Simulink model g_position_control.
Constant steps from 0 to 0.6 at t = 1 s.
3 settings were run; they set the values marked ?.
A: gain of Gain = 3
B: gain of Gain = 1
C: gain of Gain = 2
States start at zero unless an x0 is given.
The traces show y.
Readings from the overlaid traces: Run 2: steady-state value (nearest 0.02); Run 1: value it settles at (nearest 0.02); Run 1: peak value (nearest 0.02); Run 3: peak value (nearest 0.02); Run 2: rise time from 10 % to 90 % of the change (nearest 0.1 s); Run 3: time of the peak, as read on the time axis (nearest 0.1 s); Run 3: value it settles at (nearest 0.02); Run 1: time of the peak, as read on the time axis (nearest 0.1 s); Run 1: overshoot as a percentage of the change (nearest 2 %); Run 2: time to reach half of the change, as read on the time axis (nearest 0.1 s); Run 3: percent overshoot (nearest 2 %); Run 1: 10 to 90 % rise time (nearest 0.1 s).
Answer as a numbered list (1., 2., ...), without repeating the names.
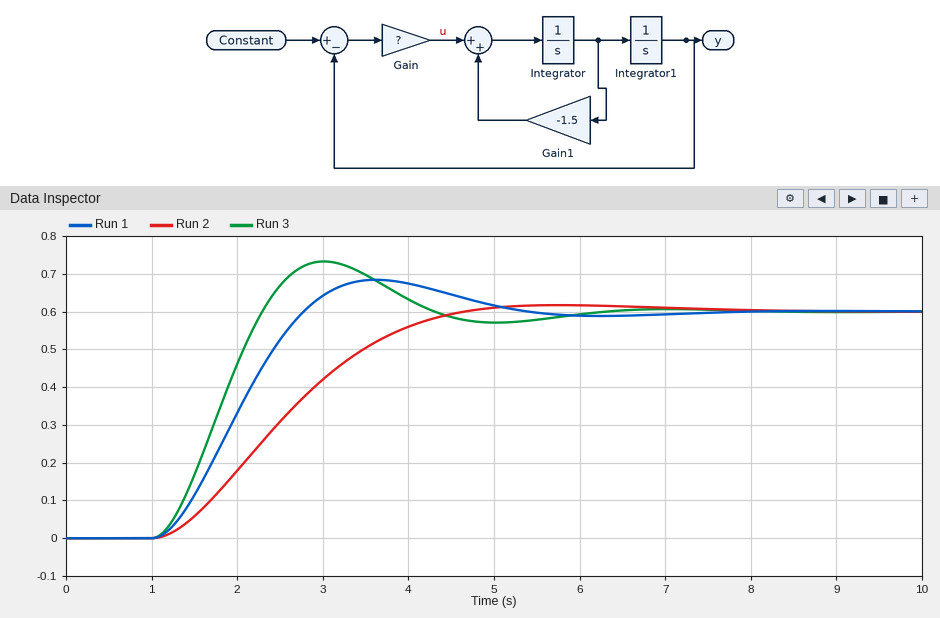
1. 0.60
2. 0.60
3. 0.68
4. 0.74
5. 2.3 s
6. 3.0 s
7. 0.60
8. 3.6 s
9. 14 %
10. 2.5 s
11. 22 %
12. 1.2 s
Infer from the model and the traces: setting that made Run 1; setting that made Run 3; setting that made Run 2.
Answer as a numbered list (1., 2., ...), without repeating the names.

1. C
2. A
3. B
